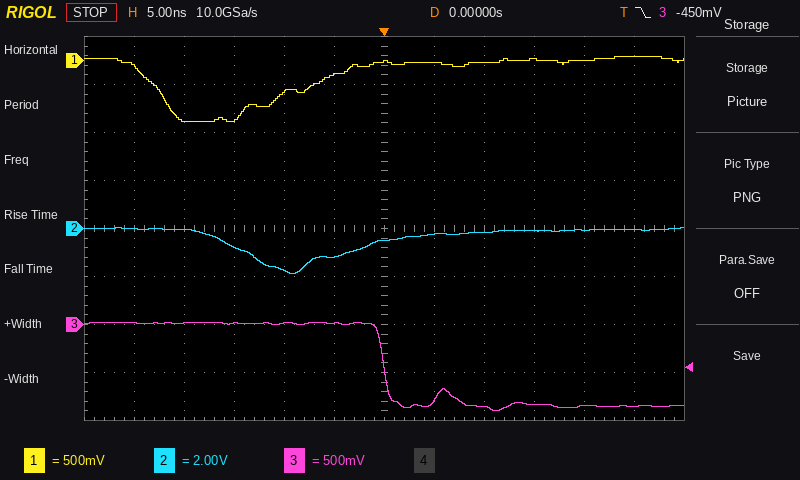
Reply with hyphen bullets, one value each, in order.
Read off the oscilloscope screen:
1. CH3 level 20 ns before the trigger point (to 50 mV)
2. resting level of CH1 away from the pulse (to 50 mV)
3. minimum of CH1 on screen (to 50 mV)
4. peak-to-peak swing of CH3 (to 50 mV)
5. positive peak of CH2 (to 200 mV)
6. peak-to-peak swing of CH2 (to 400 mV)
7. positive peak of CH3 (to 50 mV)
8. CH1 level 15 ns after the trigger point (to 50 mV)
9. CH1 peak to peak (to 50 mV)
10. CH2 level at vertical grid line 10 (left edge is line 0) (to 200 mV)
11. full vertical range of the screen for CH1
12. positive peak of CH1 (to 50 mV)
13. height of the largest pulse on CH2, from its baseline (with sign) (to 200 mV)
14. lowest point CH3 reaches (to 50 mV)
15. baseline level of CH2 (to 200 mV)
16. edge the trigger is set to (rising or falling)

- 0 mV
- 0 mV
- -650 mV
- 900 mV
- 0.0 V
- 2.0 V
- 0 mV
- 0 mV
- 700 mV
- 0.0 V
- 4 V
- 50 mV
- -1.8 V
- -900 mV
- 0.0 V
- falling
